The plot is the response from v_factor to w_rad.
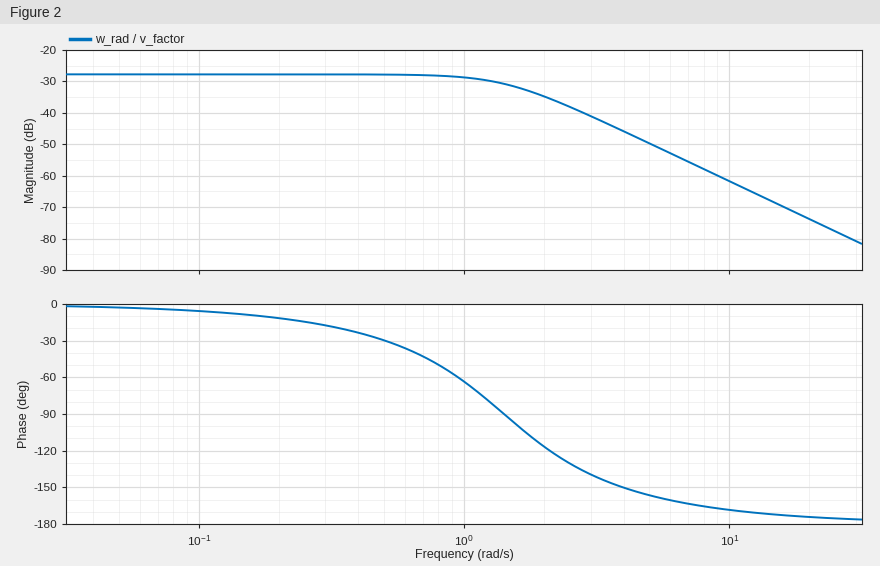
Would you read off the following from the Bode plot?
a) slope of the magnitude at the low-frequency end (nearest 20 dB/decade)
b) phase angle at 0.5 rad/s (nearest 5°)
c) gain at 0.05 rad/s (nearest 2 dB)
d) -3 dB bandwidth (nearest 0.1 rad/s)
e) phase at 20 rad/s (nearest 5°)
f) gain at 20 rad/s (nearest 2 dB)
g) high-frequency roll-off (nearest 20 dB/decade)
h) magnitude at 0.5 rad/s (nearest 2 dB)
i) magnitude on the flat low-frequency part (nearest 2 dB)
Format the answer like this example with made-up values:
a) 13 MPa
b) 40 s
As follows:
a) 0 dB/decade
b) -30°
c) -28 dB
d) 1.4 rad/s
e) -175°
f) -74 dB
g) -40 dB/decade
h) -28 dB
i) -28 dB
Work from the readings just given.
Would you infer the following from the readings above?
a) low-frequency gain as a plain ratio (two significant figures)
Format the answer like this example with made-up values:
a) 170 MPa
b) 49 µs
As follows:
a) 0.040
